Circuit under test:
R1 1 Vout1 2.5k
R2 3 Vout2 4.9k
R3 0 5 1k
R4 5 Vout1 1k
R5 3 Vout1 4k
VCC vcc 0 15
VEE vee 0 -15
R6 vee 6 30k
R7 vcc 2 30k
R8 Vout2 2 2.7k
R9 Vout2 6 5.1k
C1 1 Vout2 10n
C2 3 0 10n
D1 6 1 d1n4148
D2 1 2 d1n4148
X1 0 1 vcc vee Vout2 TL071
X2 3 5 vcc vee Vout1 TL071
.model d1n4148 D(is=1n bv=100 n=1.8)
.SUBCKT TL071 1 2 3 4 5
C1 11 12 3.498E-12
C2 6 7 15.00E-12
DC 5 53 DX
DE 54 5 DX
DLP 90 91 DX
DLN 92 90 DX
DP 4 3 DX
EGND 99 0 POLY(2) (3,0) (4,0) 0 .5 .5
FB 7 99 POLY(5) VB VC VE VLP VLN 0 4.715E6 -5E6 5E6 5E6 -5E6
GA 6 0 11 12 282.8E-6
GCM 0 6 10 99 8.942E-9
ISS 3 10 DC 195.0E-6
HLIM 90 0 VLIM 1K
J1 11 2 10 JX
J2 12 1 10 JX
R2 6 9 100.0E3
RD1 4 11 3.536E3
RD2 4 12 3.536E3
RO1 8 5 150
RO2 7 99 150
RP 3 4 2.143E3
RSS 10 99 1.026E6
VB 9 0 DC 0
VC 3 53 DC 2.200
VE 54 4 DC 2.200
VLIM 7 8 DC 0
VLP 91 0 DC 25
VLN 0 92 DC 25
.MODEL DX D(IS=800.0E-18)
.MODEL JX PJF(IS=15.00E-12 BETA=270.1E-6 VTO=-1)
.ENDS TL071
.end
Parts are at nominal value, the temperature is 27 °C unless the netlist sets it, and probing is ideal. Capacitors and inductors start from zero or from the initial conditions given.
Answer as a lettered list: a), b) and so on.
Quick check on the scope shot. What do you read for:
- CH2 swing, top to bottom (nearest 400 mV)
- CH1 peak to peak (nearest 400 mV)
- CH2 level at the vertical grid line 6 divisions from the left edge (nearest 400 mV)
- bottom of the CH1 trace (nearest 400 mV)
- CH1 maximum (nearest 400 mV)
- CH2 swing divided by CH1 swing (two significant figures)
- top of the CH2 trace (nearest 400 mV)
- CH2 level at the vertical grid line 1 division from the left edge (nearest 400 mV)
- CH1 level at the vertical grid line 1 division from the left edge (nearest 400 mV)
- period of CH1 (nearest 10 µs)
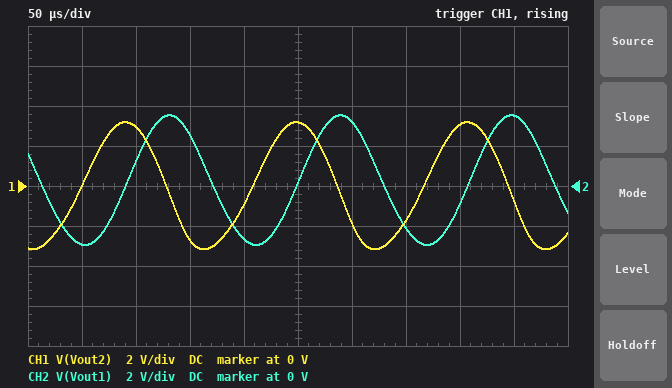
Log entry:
a) 6.4 V
b) 6.4 V
c) 3.2 V
d) -3.2 V
e) 3.2 V
f) 1.0
g) 3.6 V
h) -2.8 V
i) 0 V
j) 160 µs
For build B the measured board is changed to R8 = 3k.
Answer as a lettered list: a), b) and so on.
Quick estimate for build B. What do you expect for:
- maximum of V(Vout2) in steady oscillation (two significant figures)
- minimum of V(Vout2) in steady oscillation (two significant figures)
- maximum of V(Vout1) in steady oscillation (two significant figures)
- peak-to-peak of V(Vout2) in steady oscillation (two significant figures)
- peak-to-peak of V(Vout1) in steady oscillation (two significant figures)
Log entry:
a) 3.5 V
b) -3.5 V
c) 3.8 V
d) 7.0 V
e) 7.1 V
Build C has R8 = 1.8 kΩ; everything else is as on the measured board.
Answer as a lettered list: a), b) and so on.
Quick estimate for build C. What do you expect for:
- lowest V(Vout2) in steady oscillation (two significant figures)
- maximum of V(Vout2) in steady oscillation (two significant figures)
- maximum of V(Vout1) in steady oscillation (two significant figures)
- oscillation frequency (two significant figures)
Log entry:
a) -2.1 V
b) 2.1 V
c) 2.4 V
d) 6.3 kHz
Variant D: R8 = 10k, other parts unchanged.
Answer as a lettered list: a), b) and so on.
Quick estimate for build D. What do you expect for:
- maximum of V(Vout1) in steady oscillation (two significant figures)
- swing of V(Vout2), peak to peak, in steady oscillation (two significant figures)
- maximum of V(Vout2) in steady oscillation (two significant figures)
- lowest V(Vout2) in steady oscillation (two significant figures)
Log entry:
a) 6.7 V
b) 14 V
c) 7.2 V
d) -7.1 V
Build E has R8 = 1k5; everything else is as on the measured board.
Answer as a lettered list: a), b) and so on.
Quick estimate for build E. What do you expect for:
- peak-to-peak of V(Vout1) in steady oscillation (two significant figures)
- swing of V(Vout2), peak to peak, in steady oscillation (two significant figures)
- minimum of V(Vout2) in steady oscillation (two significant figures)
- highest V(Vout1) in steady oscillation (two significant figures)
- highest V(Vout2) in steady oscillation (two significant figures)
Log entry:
a) 3.7 V
b) 3.6 V
c) -1.8 V
d) 2.0 V
e) 1.8 V
